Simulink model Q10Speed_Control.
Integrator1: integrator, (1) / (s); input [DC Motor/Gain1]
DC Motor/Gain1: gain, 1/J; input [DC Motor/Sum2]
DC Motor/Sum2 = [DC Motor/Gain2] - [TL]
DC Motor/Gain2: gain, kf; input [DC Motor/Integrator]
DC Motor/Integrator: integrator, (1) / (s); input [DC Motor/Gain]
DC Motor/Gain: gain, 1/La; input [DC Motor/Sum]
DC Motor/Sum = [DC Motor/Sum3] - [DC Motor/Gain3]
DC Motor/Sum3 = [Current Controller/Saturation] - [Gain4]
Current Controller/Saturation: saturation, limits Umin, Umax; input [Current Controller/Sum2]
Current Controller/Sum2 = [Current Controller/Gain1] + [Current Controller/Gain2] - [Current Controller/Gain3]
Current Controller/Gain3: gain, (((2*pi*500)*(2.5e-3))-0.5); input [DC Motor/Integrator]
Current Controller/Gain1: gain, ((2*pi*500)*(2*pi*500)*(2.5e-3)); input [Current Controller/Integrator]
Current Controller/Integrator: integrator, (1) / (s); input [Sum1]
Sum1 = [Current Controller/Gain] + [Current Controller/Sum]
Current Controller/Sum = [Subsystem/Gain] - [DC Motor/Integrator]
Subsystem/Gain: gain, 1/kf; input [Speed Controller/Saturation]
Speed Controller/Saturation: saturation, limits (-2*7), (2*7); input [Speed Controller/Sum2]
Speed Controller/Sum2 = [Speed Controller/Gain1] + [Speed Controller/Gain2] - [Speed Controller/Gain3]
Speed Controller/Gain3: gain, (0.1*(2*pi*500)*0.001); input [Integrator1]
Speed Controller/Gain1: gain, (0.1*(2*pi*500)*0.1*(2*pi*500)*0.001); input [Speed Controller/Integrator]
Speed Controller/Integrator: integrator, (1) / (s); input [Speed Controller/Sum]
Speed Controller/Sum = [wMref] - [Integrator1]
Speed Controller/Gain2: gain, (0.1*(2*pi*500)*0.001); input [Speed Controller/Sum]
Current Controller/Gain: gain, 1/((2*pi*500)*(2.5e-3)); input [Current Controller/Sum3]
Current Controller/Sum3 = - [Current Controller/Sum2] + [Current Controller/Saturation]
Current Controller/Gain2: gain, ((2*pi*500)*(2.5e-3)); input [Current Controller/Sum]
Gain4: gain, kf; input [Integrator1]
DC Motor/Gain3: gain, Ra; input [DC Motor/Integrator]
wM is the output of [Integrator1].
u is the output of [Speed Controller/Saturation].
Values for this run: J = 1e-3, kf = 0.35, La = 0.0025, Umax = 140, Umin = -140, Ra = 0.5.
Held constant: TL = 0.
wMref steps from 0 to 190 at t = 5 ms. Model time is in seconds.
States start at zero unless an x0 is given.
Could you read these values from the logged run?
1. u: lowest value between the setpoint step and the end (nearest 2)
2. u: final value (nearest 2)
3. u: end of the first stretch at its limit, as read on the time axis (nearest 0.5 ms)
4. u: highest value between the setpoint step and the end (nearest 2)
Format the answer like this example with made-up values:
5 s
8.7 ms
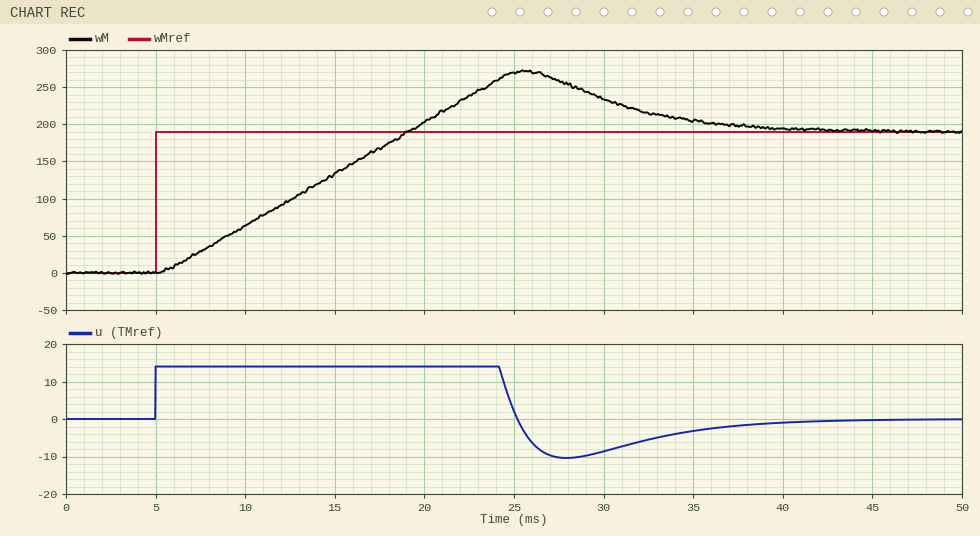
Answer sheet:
-10
0
24.0 ms
14
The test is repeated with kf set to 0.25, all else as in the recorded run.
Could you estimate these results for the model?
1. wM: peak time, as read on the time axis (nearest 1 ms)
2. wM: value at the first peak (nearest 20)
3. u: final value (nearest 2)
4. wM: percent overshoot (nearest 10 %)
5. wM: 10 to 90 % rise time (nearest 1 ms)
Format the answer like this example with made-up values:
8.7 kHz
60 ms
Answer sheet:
26 ms
280
0
40 %
11 ms
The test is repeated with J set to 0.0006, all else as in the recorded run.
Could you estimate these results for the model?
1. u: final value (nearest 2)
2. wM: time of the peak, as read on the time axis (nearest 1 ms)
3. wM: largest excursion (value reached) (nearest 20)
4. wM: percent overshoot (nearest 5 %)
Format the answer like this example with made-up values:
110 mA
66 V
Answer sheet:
0
16 ms
220
20 %
